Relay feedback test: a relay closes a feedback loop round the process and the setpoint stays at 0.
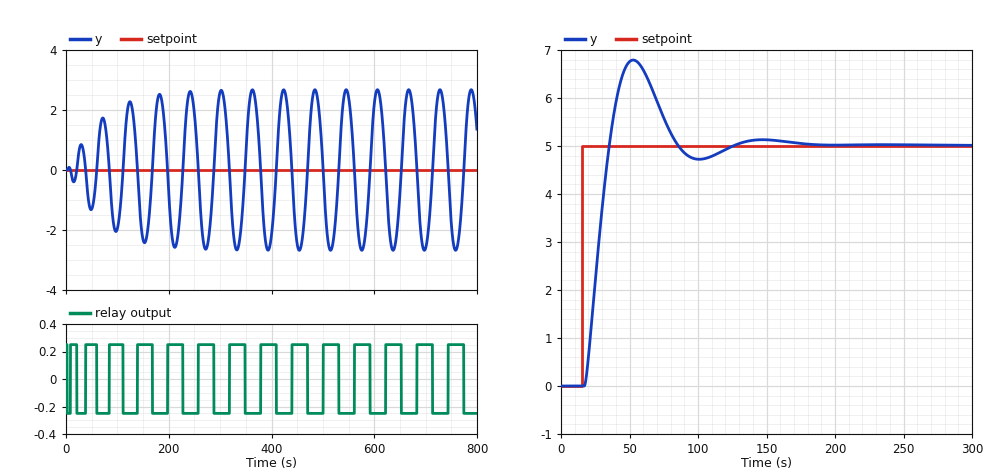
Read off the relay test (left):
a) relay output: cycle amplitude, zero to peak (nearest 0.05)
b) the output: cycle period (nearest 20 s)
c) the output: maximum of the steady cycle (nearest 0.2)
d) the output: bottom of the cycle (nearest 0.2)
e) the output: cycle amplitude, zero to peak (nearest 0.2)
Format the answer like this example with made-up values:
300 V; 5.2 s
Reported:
0.25; 60 s; 2.6; -2.6; 2.6
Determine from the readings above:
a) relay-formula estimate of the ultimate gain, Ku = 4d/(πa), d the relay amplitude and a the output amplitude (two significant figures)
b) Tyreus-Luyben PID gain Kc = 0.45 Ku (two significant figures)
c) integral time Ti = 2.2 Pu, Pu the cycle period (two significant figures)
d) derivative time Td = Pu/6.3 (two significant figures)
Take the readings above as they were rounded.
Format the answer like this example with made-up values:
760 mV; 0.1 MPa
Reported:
0.12; 0.054; 130 s; 9.5 s
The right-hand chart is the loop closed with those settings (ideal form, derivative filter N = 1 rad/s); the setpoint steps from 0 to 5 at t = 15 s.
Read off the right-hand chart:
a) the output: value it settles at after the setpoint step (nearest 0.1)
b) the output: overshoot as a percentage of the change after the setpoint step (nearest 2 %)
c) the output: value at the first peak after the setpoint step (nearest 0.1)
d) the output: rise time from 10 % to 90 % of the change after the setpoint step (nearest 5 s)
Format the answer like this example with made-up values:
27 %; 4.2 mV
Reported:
5.0; 36 %; 6.8; 15 s
